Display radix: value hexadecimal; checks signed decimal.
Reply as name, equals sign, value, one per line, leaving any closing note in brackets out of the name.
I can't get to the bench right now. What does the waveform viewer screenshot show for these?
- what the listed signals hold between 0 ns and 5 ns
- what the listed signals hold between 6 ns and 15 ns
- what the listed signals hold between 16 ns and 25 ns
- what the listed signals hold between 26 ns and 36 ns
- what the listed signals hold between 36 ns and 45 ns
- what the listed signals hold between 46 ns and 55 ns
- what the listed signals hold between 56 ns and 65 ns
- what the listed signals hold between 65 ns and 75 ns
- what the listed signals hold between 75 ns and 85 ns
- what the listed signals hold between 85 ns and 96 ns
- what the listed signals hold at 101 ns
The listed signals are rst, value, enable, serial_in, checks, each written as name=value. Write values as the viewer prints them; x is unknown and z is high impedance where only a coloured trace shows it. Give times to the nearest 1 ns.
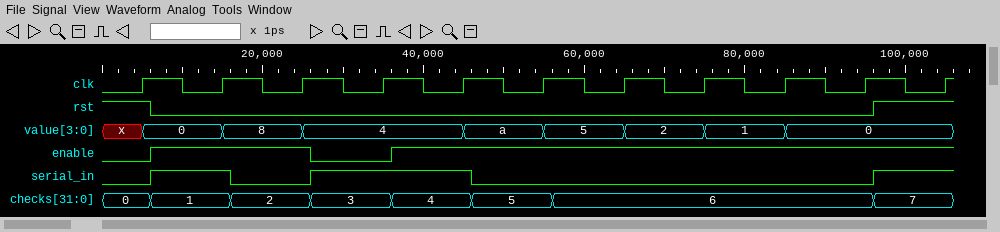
what the listed signals hold between 0 ns and 5 ns = rst=1, value=x, enable=0, serial_in=0, checks=0
what the listed signals hold between 6 ns and 15 ns = rst=0, value=0, enable=1, serial_in=1, checks=1
what the listed signals hold between 16 ns and 25 ns = rst=0, value=8, enable=1, serial_in=0, checks=2
what the listed signals hold between 26 ns and 36 ns = rst=0, value=4, enable=0, serial_in=1, checks=3
what the listed signals hold between 36 ns and 45 ns = rst=0, value=4, enable=1, serial_in=1, checks=4
what the listed signals hold between 46 ns and 55 ns = rst=0, value=a, enable=1, serial_in=0, checks=5
what the listed signals hold between 56 ns and 65 ns = rst=0, value=5, enable=1, serial_in=0, checks=6
what the listed signals hold between 65 ns and 75 ns = rst=0, value=2, enable=1, serial_in=0, checks=6
what the listed signals hold between 75 ns and 85 ns = rst=0, value=1, enable=1, serial_in=0, checks=6
what the listed signals hold between 85 ns and 96 ns = rst=0, value=0, enable=1, serial_in=0, checks=6
what the listed signals hold at 101 ns = rst=1, value=0, enable=1, serial_in=1, checks=7
